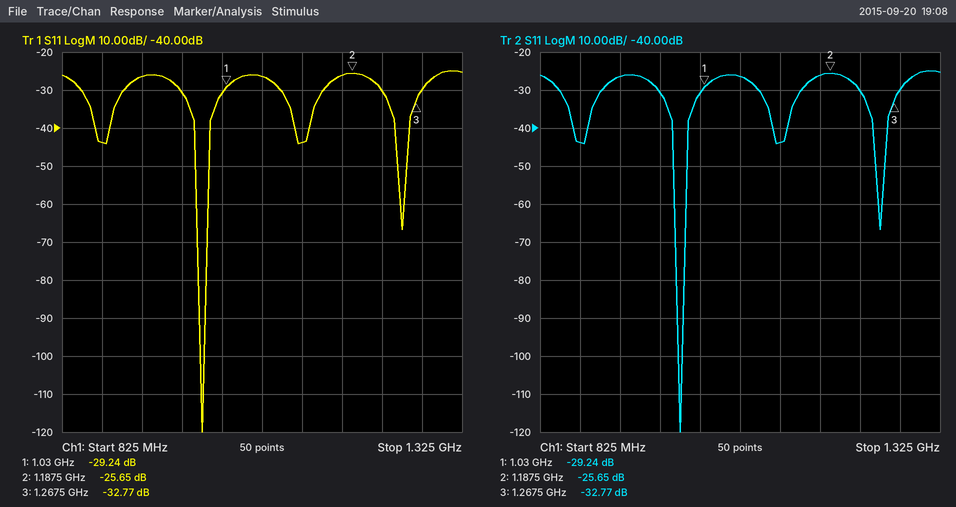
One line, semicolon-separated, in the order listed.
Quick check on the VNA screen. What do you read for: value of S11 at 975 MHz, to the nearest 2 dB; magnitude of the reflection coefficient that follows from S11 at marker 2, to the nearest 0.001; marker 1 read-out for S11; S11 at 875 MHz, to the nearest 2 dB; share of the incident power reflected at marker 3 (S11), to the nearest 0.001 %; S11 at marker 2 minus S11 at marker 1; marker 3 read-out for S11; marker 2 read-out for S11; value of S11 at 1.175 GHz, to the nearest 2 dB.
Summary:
-30 dB; 0.052; -29.24 dB; -44 dB; 0.053 %; 3.59 dB; -32.77 dB; -25.65 dB; -26 dB
